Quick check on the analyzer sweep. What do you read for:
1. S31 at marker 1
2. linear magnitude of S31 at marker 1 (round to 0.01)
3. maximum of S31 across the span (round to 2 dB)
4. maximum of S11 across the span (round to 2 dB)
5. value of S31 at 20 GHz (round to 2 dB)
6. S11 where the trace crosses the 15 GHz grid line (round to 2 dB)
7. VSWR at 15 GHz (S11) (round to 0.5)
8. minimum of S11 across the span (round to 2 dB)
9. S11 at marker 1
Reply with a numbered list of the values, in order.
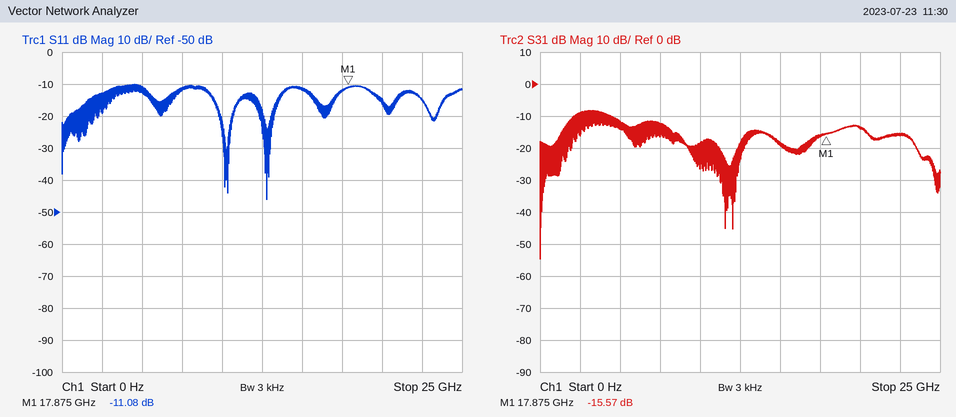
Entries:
1. -15.57 dB
2. 0.17
3. -8 dB
4. -10 dB
5. -14 dB
6. -12 dB
7. 1.5
8. -46 dB
9. -11.08 dB
